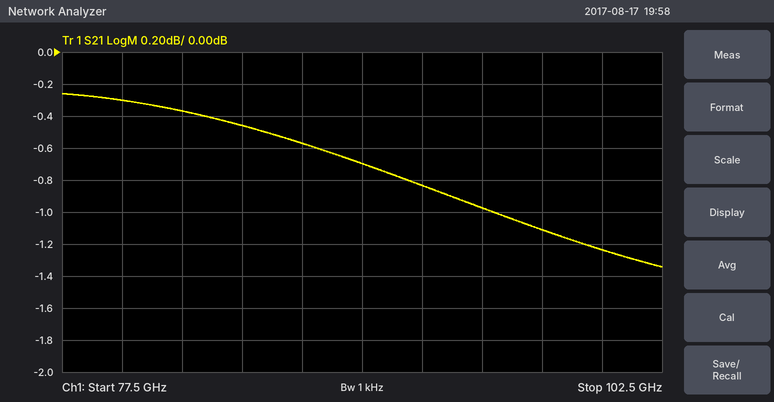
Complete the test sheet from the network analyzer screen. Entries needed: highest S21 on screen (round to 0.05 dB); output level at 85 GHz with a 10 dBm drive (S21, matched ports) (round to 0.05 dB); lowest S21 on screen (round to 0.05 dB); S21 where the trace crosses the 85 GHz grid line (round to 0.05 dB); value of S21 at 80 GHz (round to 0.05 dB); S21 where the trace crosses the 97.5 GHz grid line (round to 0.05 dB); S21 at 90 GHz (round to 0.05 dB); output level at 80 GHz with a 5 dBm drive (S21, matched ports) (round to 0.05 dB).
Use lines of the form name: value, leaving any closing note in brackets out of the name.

highest S21 on screen: -0.25 dB
output level at 85 GHz with a 10 dBm drive (S21, matched ports): 9.55 dBm
lowest S21 on screen: -1.35 dB
S21 where the trace crosses the 85 GHz grid line: -0.45 dB
value of S21 at 80 GHz: -0.30 dB
S21 where the trace crosses the 97.5 GHz grid line: -1.10 dB
S21 at 90 GHz: -0.70 dB
output level at 80 GHz with a 5 dBm drive (S21, matched ports): 4.70 dBm
